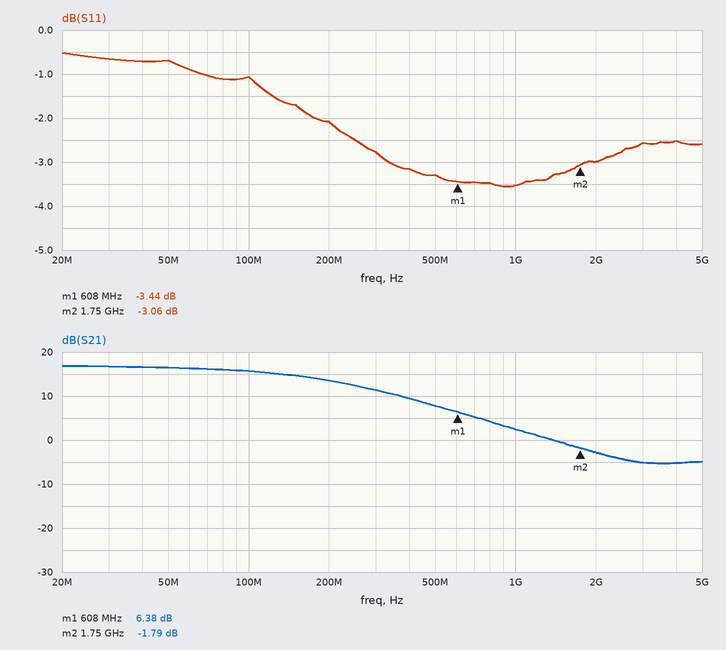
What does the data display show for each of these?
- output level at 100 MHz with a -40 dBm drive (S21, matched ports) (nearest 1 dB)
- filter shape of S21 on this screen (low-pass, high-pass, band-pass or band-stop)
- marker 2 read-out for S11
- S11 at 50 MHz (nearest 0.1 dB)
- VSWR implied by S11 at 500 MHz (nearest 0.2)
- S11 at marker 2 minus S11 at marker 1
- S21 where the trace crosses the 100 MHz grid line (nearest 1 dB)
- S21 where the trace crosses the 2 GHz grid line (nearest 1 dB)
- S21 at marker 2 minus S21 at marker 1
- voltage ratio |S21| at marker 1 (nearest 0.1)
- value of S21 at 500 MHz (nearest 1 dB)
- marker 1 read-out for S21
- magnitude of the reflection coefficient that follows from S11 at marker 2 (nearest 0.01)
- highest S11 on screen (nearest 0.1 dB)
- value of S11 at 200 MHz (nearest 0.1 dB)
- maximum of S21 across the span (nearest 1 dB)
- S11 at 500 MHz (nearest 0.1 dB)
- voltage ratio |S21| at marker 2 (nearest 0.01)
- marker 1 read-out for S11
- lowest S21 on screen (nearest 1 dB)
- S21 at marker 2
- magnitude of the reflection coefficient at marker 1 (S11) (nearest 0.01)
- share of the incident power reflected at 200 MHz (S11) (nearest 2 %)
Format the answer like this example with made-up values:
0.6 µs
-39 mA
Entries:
-24 dBm
low-pass
-3.06 dB
-0.7 dB
5.4
0.38 dB
16 dB
-3 dB
-8.17 dB
2.1
8 dB
6.38 dB
0.70
-0.5 dB
-2.1 dB
17 dB
-3.3 dB
0.81
-3.44 dB
-5 dB
-1.79 dB
0.67
62 %
